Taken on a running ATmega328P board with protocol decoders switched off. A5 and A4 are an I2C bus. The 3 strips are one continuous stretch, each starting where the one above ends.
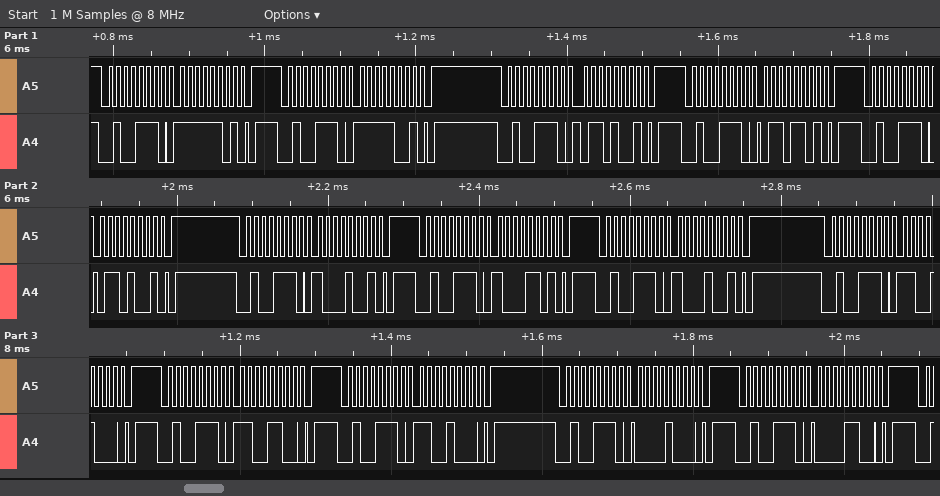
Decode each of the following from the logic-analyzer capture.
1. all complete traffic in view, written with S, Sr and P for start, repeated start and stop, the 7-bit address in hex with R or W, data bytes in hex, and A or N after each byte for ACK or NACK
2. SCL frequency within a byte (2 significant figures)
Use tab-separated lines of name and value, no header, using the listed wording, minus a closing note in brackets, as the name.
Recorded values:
all complete traffic in view, written with S, Sr and P for start, repeated start and stop, the 7-bit address in hex with R or W, data bytes in hex, and A or N after each byte for ACK or NACK	S 27W A FD A P S 27W A F9 A P S 27W A 69 A P S 27W A 6D A P S 27W A 69 A P S 27W A 89 A P S 27W A 8D A P S 27W A 89 A P S 27W A C8 A P S 27W A CC A P S 27W A C8 A P S 27W A 08 A P S 27W A 0C A P
SCL frequency within a byte	100 kHz
